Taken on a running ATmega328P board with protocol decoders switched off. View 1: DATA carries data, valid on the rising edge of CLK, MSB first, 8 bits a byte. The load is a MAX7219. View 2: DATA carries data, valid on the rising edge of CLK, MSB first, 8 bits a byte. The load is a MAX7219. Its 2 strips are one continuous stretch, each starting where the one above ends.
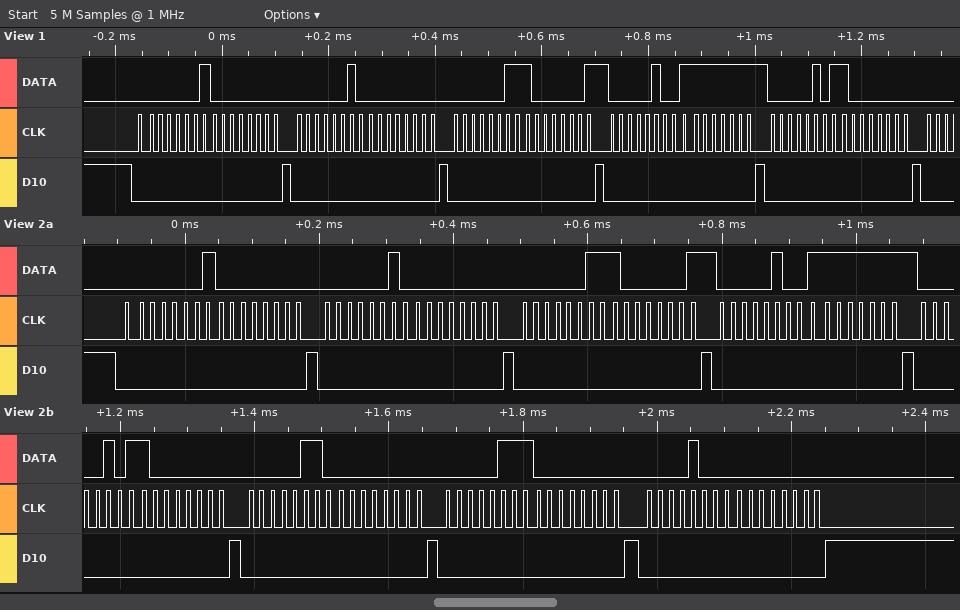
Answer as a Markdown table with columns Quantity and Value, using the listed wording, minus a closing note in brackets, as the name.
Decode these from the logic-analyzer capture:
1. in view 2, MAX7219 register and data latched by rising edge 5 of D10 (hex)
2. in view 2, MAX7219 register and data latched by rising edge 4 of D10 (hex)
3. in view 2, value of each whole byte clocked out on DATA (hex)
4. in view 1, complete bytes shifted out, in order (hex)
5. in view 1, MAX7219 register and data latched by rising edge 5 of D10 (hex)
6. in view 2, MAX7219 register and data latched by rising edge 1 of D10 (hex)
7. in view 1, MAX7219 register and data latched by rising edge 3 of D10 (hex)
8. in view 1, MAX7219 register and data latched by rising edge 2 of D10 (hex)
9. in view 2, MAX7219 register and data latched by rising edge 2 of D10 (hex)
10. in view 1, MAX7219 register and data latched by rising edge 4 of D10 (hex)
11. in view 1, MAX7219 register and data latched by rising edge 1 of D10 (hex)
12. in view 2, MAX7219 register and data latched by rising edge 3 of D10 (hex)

| Quantity | Value |
|---|---|
| in view 2, MAX7219 register and data latched by rising edge 5 of D10 | register 0x5, data 0x80 |
| in view 2, MAX7219 register and data latched by rising edge 4 of D10 | register 0x4, data 0xFF |
| in view 2, value of each whole byte clocked out on DATA | 01 00 02 00 03 81 04 FF 05 80 06 00 07 00 08 00 |
| in view 1, complete bytes shifted out, in order | 01 00 02 00 03 81 04 FF 05 80 |
| in view 1, MAX7219 register and data latched by rising edge 5 of D10 | register 0x5, data 0x80 |
| in view 2, MAX7219 register and data latched by rising edge 1 of D10 | register 0x1, data 0x00 |
| in view 1, MAX7219 register and data latched by rising edge 3 of D10 | register 0x3, data 0x81 |
| in view 1, MAX7219 register and data latched by rising edge 2 of D10 | register 0x2, data 0x00 |
| in view 2, MAX7219 register and data latched by rising edge 2 of D10 | register 0x2, data 0x00 |
| in view 1, MAX7219 register and data latched by rising edge 4 of D10 | register 0x4, data 0xFF |
| in view 1, MAX7219 register and data latched by rising edge 1 of D10 | register 0x1, data 0x00 |
| in view 2, MAX7219 register and data latched by rising edge 3 of D10 | register 0x3, data 0x81 |
